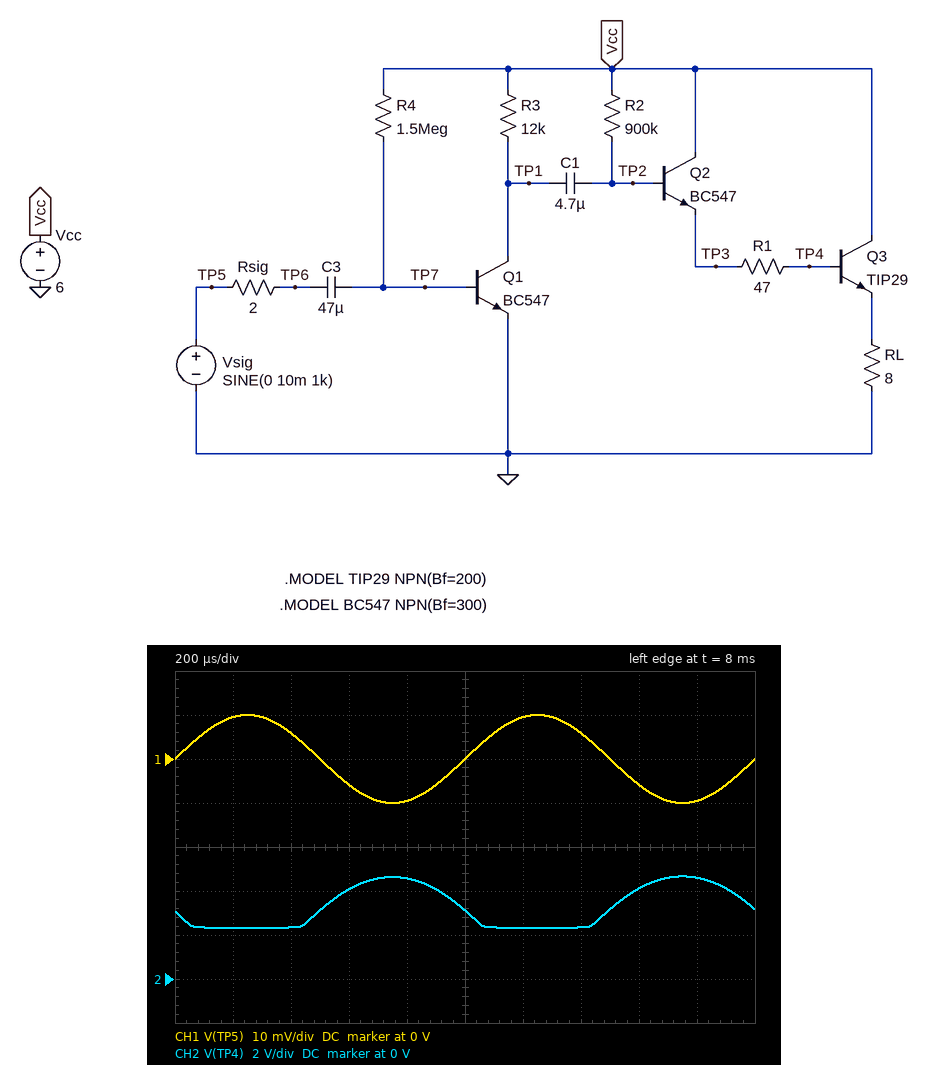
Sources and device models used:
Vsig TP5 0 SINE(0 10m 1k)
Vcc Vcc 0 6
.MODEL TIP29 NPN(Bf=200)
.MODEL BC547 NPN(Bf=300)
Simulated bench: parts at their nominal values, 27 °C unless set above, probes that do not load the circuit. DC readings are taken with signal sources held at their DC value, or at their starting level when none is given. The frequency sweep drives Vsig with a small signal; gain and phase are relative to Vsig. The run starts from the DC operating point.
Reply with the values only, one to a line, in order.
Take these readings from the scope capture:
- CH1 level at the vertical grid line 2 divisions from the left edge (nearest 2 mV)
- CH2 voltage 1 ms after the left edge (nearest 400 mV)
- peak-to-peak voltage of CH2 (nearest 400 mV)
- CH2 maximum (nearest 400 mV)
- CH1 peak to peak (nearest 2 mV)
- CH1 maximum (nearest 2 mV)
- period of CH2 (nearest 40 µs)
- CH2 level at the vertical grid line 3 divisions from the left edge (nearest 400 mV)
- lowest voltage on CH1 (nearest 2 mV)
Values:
6 mV
3.2 V
2.4 V
4.8 V
20 mV
10 mV
1.00 ms
4.0 V
-10 mV
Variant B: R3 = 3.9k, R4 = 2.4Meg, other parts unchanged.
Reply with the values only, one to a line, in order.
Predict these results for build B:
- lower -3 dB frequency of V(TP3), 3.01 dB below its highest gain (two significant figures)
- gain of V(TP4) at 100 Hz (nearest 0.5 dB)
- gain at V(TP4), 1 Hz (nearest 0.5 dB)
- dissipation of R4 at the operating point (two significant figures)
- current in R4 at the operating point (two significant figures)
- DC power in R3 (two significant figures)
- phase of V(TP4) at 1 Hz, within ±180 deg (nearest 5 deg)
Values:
320 mHz
39.5 dB
39.0 dB
11 µW
2.2 µA
1.7 mW
-160 deg
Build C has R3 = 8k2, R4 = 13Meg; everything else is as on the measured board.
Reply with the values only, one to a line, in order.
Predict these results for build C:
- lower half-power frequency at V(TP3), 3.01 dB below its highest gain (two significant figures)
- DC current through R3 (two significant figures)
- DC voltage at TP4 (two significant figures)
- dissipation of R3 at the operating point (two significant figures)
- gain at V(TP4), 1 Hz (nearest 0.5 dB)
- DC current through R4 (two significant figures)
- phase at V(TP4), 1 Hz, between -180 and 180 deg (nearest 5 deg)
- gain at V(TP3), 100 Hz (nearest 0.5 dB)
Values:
120 mHz
120 µA
2.4 V
120 µW
31.0 dB
410 nA
-170 deg
31.5 dB
